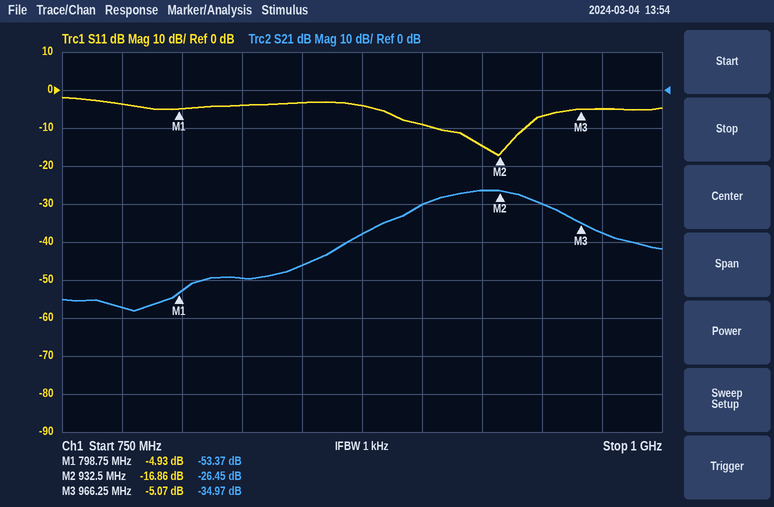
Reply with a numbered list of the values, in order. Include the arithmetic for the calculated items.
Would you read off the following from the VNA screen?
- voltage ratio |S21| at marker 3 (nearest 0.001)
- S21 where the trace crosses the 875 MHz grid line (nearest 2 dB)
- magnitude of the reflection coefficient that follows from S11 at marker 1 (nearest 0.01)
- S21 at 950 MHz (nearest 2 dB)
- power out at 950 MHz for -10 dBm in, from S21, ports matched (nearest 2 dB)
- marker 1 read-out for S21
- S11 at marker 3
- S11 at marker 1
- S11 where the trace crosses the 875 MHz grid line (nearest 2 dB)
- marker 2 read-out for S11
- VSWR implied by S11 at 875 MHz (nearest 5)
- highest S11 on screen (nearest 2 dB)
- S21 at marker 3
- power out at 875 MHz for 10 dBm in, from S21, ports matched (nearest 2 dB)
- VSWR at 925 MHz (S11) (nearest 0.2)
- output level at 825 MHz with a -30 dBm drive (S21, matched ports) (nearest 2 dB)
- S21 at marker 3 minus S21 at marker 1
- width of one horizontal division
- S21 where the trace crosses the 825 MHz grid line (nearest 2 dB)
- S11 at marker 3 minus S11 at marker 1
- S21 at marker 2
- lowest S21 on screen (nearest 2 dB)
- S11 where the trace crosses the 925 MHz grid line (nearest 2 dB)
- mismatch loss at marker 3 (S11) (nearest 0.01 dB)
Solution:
1. 10^(-34.97/20) ≈ 0.018
2. -38 dB
3. 10^(-4.93/20) ≈ 0.57
4. -30 dB
5. -10 dBm + (-30 dB) = -40 dBm
6. -53.37 dB
7. -5.07 dB
8. -4.93 dB
9. -4 dB
10. -16.86 dB
11. |Γ| = 10^(-4/20) = 0.6310; VSWR = (1 + 0.6310)/(1 − 0.6310) ≈ 4.42, so 5 to the nearest 5
12. -2 dB
13. -34.97 dB
14. 10 dBm + (-38 dB) = -28 dBm
15. |Γ| = 10^(-14/20) = 0.1995; VSWR = (1 + 0.1995)/(1 − 0.1995) ≈ 1.50, so 1.4 to the nearest 0.2
16. -30 dBm + (-50 dB) = -80 dBm
17. -34.97 − (-53.37) = 18.40 dB
18. 25 MHz
19. -50 dB
20. -5.07 − (-4.93) = -0.14 dB
21. -26.45 dB
22. -58 dB
23. -14 dB
24. −10 log10(1 − 10^(-5.07/10)) ≈ 1.62 dB
